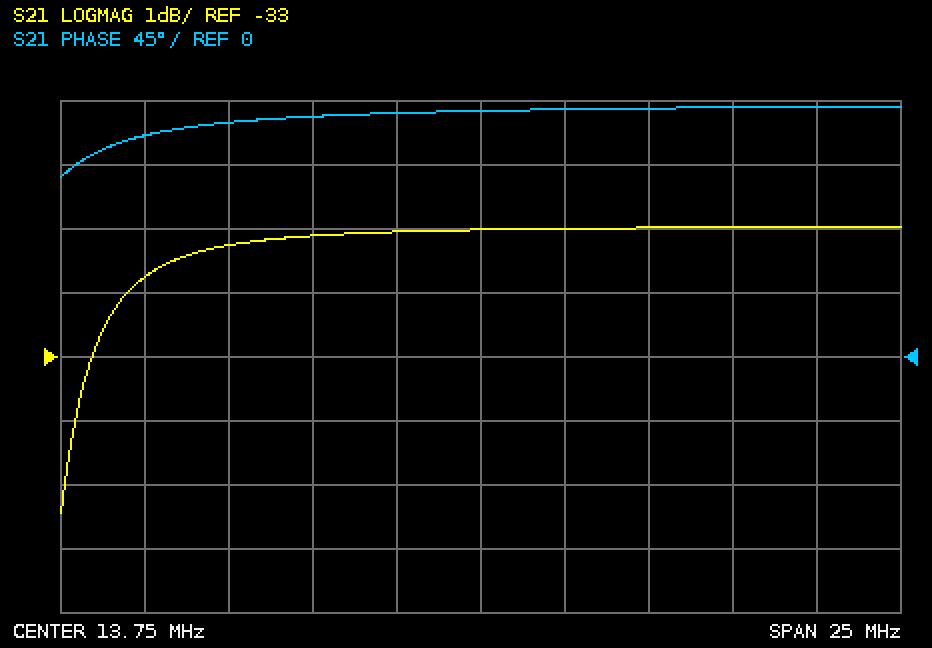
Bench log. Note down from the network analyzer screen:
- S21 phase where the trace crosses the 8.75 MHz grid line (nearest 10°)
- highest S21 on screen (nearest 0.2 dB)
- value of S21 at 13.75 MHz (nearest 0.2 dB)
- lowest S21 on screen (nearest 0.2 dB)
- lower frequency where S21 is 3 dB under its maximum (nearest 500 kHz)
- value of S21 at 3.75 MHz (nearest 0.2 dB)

170°
-31.0 dB
-31.0 dB
-35.4 dB
1.5 MHz
-31.8 dB
